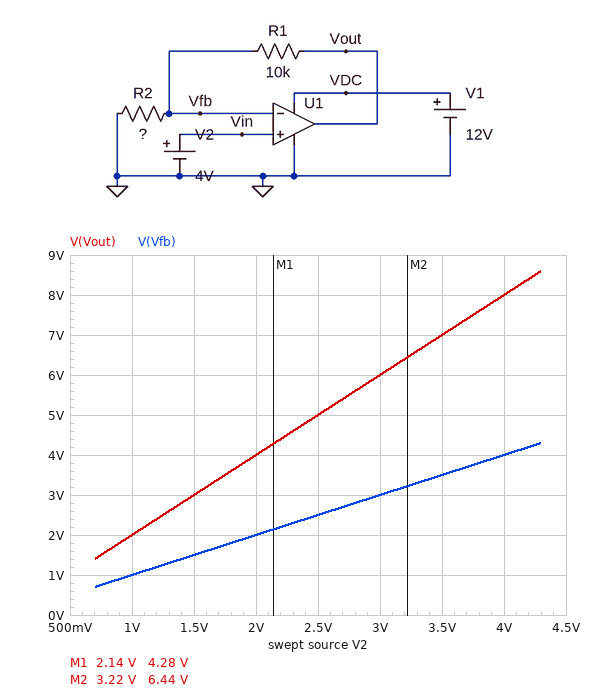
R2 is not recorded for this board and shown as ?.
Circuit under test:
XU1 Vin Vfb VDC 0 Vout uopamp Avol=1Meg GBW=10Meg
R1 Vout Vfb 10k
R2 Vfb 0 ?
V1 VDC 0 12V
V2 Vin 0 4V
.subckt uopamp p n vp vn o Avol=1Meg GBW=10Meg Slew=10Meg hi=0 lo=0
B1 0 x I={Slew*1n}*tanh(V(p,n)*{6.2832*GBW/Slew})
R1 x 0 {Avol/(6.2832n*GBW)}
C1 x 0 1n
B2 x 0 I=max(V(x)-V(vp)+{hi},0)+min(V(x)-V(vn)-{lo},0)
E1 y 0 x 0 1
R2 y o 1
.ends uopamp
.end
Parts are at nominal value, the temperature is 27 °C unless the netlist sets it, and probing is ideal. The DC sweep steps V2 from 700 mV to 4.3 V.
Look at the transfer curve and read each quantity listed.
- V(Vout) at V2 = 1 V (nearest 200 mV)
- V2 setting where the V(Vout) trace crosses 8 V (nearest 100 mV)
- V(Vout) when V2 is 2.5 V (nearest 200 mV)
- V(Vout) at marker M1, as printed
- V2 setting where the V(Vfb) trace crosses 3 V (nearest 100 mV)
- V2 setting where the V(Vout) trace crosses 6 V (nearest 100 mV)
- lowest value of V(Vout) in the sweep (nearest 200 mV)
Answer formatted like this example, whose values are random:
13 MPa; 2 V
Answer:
2.0 V; 4.0 V; 5.0 V; 4.28 V; 3.0 V; 3.0 V; 1.4 V
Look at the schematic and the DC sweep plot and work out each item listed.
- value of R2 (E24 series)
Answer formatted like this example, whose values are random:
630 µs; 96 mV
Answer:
10 kΩ
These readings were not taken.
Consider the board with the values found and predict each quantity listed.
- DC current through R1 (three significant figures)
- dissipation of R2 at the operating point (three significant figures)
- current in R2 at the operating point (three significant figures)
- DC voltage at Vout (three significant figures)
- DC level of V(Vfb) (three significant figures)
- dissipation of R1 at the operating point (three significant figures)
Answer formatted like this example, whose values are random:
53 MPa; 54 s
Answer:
400 µA; 1.60 mW; 400 µA; 8.00 V; 4.00 V; 1.60 mW
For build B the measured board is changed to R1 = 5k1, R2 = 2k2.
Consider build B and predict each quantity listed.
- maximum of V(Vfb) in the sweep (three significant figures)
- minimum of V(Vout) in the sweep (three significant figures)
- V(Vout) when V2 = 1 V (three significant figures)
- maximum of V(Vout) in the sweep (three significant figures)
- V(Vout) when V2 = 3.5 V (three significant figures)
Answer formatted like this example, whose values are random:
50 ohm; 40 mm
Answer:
3.62 V; 2.32 V; 3.32 V; 12.0 V; 11.6 V
